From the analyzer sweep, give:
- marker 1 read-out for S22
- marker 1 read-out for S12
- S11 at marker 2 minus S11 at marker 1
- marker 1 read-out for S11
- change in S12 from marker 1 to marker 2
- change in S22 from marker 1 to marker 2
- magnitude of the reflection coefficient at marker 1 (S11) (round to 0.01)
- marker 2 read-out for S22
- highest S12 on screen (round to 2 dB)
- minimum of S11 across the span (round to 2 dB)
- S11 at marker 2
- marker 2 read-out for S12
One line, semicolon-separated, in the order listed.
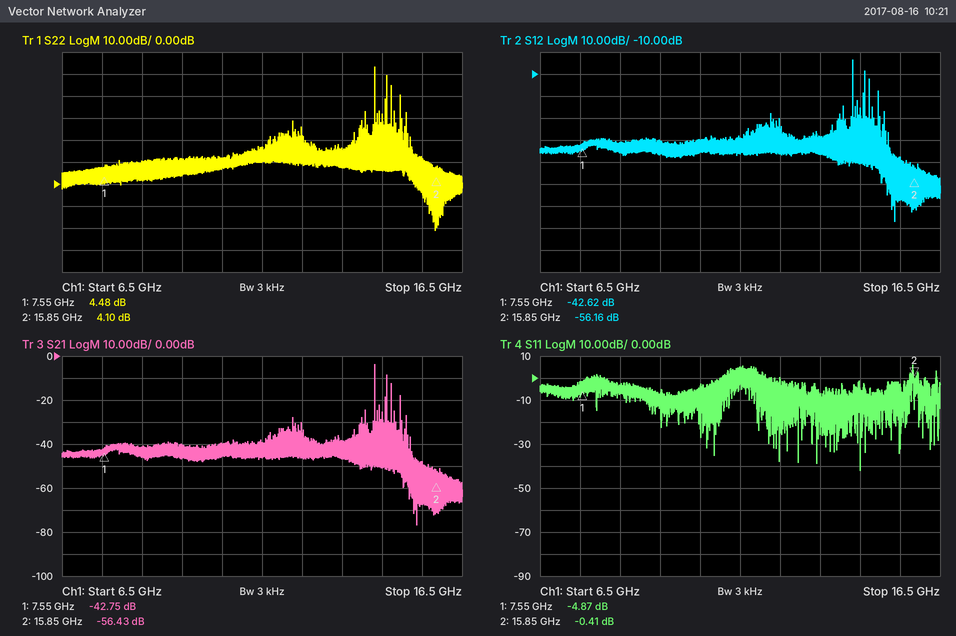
4.48 dB; -42.62 dB; 4.46 dB; -4.87 dB; -13.54 dB; -0.38 dB; 0.57; 4.10 dB; -4 dB; -42 dB; -0.41 dB; -56.16 dB
